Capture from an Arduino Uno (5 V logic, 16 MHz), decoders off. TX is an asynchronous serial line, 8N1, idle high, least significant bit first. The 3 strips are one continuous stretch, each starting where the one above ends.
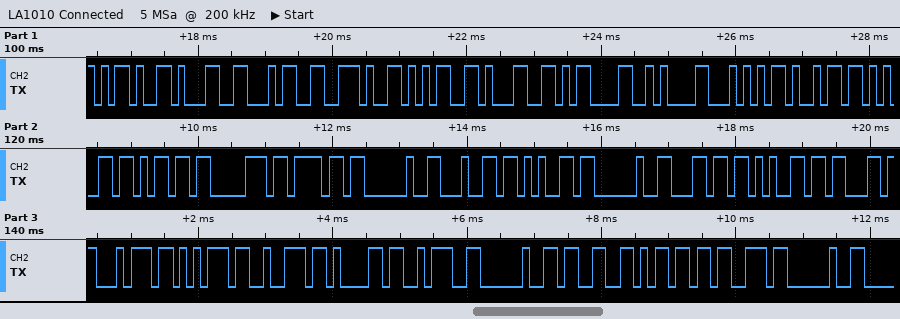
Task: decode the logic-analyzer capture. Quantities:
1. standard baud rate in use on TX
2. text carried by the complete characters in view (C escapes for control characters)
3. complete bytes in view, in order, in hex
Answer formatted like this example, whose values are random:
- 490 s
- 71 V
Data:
- 9600 baud
- "-14.51\r\nTiempo de lectura: 3ms "
- 2D 31 34 2E 35 31 0D 0A 54 69 65 6D 70 6F 20 64 65 20 6C 65 63 74 75 72 61 3A 20 33 6D 73 20
